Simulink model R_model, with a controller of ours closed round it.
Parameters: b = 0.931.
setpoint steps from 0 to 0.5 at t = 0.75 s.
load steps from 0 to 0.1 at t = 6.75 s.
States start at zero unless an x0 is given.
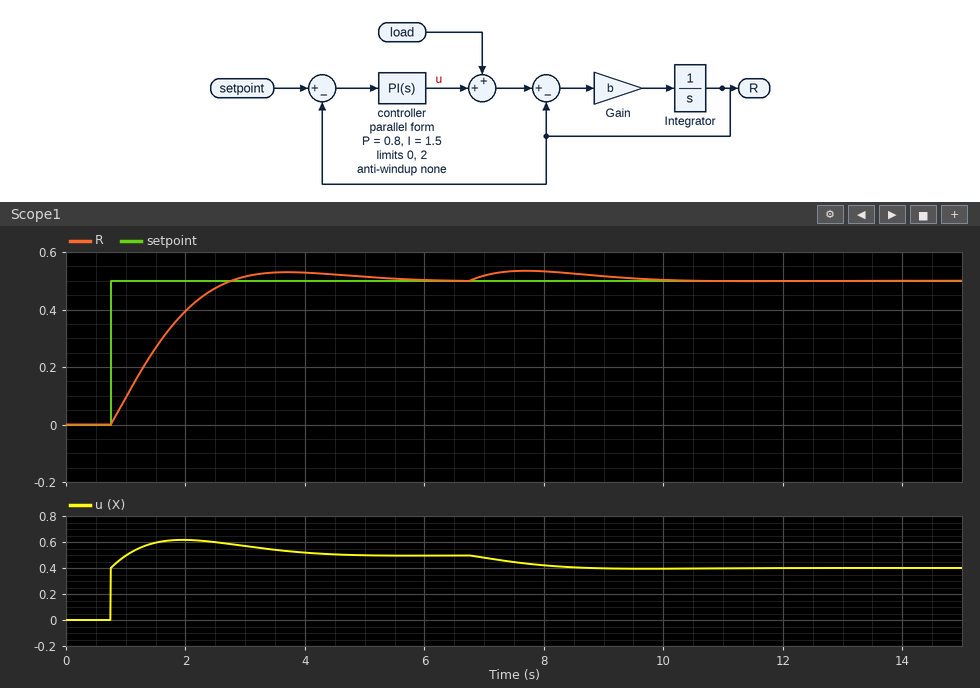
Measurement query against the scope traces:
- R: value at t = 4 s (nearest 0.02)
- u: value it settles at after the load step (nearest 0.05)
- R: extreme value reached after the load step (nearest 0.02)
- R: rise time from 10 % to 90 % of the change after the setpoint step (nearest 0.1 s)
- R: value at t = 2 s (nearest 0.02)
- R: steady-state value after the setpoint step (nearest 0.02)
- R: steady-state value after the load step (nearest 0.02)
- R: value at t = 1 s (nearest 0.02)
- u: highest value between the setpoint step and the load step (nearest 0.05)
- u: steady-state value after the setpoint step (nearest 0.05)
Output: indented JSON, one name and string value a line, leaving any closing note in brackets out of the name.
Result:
{
  "R: value at t = 4 s": "0.52",
  "u: value it settles at after the load step": "0.40",
  "R: extreme value reached after the load step": "0.54",
  "R: rise time from 10 % to 90 % of the change after the setpoint step": "1.4 s",
  "R: value at t = 2 s": "0.40",
  "R: steady-state value after the setpoint step": "0.50",
  "R: steady-state value after the load step": "0.50",
  "R: value at t = 1 s": "0.10",
  "u: highest value between the setpoint step and the load step": "0.60",
  "u: steady-state value after the setpoint step": "0.50"
}
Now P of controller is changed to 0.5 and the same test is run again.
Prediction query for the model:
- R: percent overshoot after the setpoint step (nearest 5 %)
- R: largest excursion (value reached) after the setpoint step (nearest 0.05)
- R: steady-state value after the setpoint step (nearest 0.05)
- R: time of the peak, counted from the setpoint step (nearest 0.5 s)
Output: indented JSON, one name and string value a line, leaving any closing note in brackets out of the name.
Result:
{
  "R: percent overshoot after the setpoint step": "10 %",
  "R: largest excursion (value reached) after the setpoint step": "0.55",
  "R: steady-state value after the setpoint step": "0.50",
  "R: time of the peak, counted from the setpoint step": "3.0 s"
}
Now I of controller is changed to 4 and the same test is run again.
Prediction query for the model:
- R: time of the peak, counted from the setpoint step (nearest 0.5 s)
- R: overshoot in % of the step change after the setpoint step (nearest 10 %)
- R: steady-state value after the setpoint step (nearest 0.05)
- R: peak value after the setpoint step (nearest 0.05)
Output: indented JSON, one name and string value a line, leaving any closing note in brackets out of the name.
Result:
{
  "R: time of the peak, counted from the setpoint step": "1.5 s",
  "R: overshoot in % of the step change after the setpoint step": "20 %",
  "R: steady-state value after the setpoint step": "0.50",
  "R: peak value after the setpoint step": "0.60"
}
